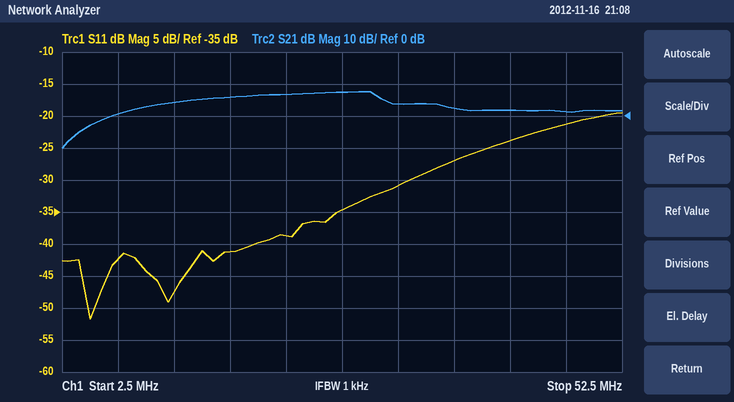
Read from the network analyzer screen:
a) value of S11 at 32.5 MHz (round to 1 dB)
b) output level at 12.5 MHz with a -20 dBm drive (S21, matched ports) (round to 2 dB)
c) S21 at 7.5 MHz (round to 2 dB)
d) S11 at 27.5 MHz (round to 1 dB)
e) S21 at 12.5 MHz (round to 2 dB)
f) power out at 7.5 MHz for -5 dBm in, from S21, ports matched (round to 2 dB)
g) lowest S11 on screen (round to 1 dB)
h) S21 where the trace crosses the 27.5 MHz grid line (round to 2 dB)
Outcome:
-31 dB
-16 dBm
0 dB
-35 dB
4 dB
-4 dBm
-52 dB
8 dB
